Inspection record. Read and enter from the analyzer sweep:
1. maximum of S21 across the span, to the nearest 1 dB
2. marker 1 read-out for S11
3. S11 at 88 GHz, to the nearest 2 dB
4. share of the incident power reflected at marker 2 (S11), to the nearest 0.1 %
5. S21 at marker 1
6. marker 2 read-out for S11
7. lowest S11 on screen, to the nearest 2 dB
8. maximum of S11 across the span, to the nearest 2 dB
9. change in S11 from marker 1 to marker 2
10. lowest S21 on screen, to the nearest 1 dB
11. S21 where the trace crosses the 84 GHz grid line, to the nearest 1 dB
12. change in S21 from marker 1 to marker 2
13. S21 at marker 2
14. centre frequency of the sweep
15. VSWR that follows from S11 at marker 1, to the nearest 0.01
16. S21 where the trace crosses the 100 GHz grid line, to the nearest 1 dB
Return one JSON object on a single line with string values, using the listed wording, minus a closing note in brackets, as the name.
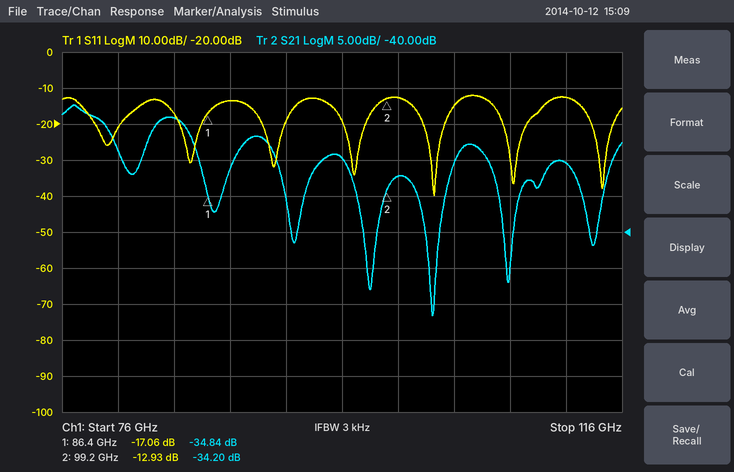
{"maximum of S21 across the span, to the nearest 1 dB": "-22 dB", "marker 1 read-out for S11": "-17.06 dB", "S11 at 88 GHz, to the nearest 2 dB": "-14 dB", "share of the incident power reflected at marker 2 (S11), to the nearest 0.1 %": "5.1 %", "S21 at marker 1": "-34.84 dB", "marker 2 read-out for S11": "-12.93 dB", "lowest S11 on screen, to the nearest 2 dB": "-40 dB", "maximum of S11 across the span, to the nearest 2 dB": "-12 dB", "change in S11 from marker 1 to marker 2": "4.13 dB", "lowest S21 on screen, to the nearest 1 dB": "-52 dB", "S21 where the trace crosses the 84 GHz grid line, to the nearest 1 dB": "-24 dB", "change in S21 from marker 1 to marker 2": "0.64 dB", "S21 at marker 2": "-34.20 dB", "centre frequency of the sweep": "96 GHz", "VSWR that follows from S11 at marker 1, to the nearest 0.01": "1.33", "S21 where the trace crosses the 100 GHz grid line, to the nearest 1 dB": "-32 dB"}
